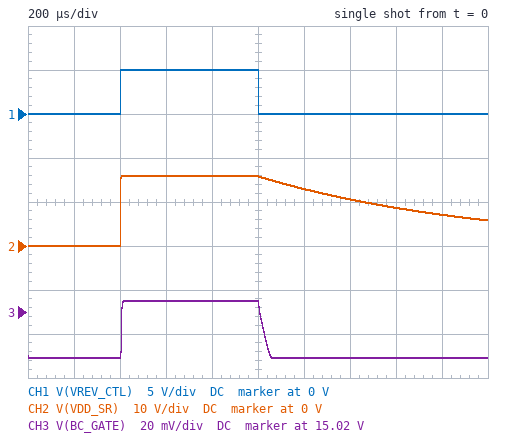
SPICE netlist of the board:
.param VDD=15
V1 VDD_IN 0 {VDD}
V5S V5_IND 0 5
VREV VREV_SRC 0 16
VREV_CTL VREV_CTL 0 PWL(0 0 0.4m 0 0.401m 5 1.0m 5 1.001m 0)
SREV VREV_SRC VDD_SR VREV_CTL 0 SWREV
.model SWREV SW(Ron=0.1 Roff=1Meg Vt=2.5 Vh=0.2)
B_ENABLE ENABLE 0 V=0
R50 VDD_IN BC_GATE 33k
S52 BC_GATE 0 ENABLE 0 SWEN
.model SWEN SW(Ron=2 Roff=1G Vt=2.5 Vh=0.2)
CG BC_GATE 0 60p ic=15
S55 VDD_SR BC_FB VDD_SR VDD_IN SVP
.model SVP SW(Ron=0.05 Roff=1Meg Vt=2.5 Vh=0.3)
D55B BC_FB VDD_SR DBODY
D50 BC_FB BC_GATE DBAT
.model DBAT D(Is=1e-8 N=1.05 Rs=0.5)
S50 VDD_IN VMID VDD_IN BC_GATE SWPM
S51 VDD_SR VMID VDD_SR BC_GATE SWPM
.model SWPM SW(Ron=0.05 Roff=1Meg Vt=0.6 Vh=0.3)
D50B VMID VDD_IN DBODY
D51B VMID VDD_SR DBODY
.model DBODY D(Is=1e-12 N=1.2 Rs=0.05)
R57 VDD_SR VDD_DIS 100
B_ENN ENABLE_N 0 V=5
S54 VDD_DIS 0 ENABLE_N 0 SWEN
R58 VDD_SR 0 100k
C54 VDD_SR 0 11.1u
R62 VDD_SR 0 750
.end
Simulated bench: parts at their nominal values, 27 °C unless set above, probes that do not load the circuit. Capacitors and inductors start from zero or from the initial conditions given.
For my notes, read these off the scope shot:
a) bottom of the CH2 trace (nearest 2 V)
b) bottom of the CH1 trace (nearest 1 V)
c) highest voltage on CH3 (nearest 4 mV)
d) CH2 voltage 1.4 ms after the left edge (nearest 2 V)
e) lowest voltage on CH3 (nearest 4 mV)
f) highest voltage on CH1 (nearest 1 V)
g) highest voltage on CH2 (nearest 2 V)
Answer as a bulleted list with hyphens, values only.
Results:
- 0 V
- 0 V
- 15.024 V
- 10 V
- 15.000 V
- 5 V
- 16 V
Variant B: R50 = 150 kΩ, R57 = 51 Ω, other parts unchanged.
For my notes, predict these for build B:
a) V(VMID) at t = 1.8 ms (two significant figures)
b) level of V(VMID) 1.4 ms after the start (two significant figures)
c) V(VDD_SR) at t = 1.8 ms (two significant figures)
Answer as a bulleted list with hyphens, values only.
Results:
- 4.2 V
- 8.1 V
- 3.7 V
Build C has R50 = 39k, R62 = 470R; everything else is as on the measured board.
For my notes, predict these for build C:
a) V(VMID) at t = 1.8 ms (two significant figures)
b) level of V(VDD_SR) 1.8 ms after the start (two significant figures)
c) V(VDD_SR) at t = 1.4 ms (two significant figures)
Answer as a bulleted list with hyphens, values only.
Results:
- 7.2 V
- 6.7 V
- 10 V
